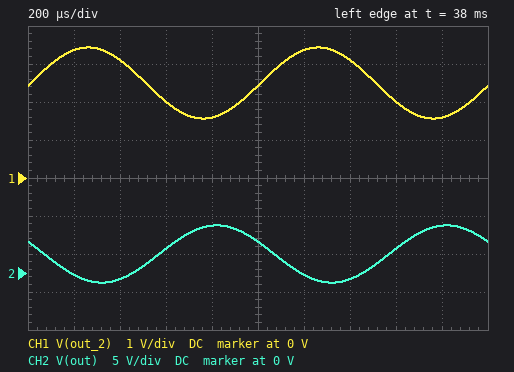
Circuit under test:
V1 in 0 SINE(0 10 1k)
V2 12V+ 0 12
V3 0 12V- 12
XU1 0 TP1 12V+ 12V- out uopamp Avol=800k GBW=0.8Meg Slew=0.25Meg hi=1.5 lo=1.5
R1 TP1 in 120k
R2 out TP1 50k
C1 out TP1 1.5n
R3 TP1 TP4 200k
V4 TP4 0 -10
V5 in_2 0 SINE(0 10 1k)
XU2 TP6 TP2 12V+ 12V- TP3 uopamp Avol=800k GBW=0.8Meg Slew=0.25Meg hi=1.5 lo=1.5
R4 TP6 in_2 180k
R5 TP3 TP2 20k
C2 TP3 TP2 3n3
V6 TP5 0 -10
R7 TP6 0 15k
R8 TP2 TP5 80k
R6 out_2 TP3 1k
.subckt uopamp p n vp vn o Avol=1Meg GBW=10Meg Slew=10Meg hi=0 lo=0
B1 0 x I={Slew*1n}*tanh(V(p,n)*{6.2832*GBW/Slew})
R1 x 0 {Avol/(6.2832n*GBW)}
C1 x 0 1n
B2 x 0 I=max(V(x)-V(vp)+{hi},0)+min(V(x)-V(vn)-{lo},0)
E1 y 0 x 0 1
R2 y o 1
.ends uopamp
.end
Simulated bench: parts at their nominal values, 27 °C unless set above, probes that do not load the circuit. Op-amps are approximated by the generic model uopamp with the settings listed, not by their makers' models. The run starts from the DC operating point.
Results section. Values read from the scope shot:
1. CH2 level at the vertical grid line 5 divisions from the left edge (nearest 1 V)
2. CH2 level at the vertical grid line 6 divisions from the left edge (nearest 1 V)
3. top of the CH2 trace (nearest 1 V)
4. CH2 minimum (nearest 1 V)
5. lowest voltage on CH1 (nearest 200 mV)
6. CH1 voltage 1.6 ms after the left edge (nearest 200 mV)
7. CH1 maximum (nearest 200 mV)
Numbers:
4 V
0 V
6 V
-1 V
1.6 V
2.0 V
3.4 V
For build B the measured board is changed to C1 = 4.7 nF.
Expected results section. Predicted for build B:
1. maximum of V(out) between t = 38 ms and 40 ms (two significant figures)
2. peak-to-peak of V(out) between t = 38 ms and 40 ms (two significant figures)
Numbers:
4.8 V
4.7 V
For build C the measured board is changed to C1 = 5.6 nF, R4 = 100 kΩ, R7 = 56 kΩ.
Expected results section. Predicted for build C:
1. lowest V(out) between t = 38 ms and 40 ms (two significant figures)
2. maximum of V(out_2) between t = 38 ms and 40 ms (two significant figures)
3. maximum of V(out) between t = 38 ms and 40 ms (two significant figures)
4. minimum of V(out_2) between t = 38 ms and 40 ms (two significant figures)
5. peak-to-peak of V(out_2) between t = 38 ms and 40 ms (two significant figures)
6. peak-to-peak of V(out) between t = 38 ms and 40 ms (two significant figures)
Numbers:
440 mV
6.9 V
4.6 V
-1.9 V
8.7 V
4.1 V
